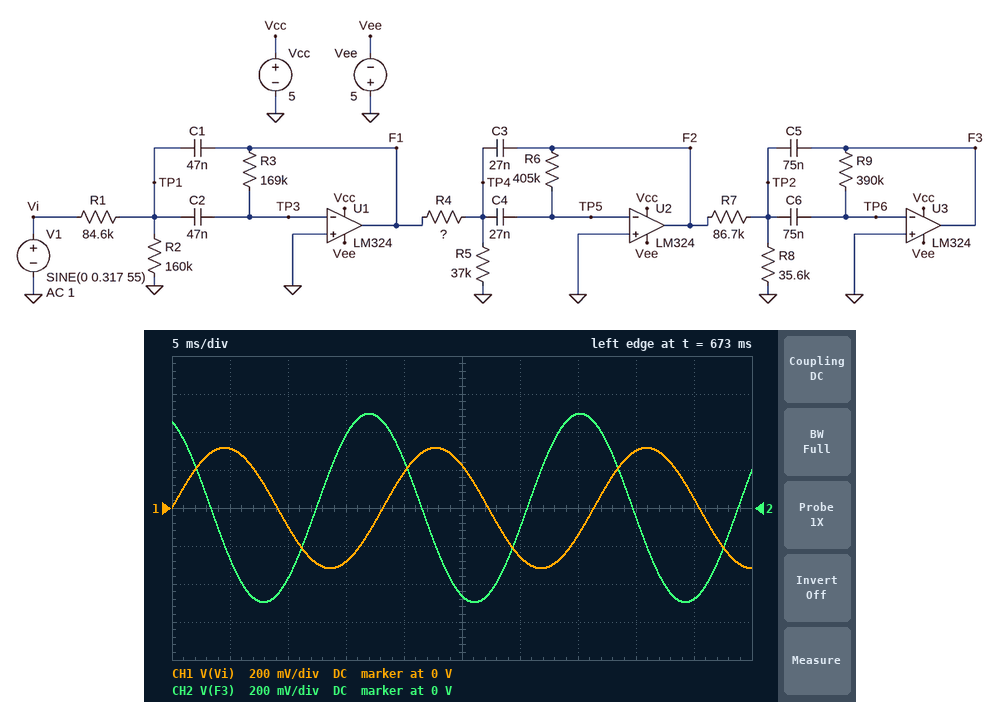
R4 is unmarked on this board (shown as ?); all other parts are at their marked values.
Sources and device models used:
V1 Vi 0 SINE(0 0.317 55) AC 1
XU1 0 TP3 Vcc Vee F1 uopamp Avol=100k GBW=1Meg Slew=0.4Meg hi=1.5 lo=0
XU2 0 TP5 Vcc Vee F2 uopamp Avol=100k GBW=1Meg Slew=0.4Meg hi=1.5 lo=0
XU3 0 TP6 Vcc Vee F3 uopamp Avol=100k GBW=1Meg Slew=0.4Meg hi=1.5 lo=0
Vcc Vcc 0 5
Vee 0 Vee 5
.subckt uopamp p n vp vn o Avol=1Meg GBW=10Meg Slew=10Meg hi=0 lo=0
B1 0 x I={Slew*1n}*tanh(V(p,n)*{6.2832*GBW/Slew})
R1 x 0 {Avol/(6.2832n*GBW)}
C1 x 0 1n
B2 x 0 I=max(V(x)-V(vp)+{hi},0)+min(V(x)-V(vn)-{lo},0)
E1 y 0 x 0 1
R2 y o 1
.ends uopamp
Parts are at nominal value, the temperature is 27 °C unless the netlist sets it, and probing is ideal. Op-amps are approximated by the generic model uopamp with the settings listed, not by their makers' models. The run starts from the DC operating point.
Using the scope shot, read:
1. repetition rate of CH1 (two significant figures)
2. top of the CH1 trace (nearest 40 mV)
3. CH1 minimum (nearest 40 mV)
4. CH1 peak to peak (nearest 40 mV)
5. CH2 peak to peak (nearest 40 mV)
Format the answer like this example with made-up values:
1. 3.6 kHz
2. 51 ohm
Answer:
1. 55 Hz
2. 320 mV
3. -320 mV
4. 640 mV
5. 1.00 V
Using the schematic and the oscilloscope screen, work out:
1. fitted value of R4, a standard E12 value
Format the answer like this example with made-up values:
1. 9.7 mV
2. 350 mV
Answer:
1. 33 kΩ
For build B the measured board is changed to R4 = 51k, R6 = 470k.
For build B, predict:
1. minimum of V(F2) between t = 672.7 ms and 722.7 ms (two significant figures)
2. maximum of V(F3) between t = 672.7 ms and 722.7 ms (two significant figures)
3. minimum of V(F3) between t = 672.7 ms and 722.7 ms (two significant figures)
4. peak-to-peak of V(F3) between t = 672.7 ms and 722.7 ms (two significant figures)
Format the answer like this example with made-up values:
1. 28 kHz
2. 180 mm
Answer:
1. -1.1 V
2. 550 mV
3. -550 mV
4. 1.1 V
